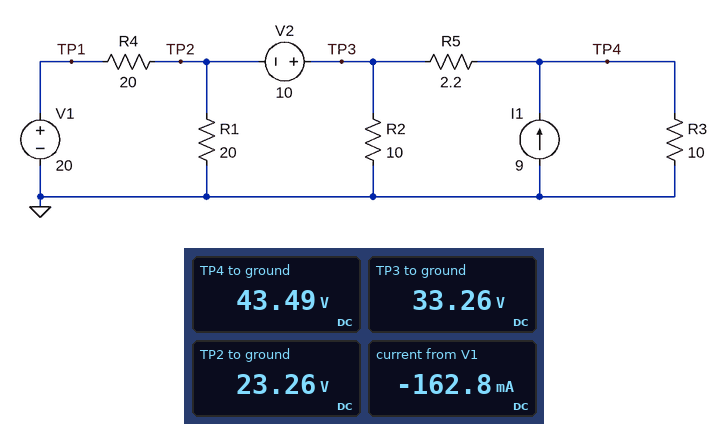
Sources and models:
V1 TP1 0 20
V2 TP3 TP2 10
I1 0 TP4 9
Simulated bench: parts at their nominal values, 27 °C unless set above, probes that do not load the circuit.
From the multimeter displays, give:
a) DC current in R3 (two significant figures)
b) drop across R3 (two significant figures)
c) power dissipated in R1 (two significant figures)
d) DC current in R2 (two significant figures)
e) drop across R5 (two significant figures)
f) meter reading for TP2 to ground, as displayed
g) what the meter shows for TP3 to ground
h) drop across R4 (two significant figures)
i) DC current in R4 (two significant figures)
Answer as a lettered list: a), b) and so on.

a) 4.3 A
b) 43 V
c) 27 W
d) 3.3 A
e) 10 V
f) 23.26 V
g) 33.26 V
h) 3.3 V
i) 160 mA
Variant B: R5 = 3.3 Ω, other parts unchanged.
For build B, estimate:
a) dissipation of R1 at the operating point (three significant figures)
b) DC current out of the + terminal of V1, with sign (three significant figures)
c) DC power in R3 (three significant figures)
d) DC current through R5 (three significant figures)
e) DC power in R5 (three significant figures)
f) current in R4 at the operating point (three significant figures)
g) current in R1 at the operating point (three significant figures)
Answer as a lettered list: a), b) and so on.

a) 23.9 W
b) -92.9 mA
c) 214 W
d) 4.37 A
e) 63.1 W
f) 92.9 mA
g) 1.09 A
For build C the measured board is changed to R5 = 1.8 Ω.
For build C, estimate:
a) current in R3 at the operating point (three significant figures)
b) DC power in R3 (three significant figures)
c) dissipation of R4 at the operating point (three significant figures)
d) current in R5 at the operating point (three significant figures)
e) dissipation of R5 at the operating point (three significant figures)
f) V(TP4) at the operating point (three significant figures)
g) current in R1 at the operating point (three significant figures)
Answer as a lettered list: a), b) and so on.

a) 4.24 A
b) 180 W
c) 726 mW
d) 4.76 A
e) 40.8 W
f) 42.4 V
g) 1.19 A
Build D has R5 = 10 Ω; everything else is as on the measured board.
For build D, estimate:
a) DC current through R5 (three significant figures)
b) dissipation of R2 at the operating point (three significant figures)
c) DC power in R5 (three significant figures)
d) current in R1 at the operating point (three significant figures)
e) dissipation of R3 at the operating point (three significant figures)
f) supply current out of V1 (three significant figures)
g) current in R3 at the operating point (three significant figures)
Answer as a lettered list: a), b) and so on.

a) 3.20 A
b) 67.6 W
c) 102 W
d) 800 mA
e) 336 W
f) 200 mA
g) 5.80 A
